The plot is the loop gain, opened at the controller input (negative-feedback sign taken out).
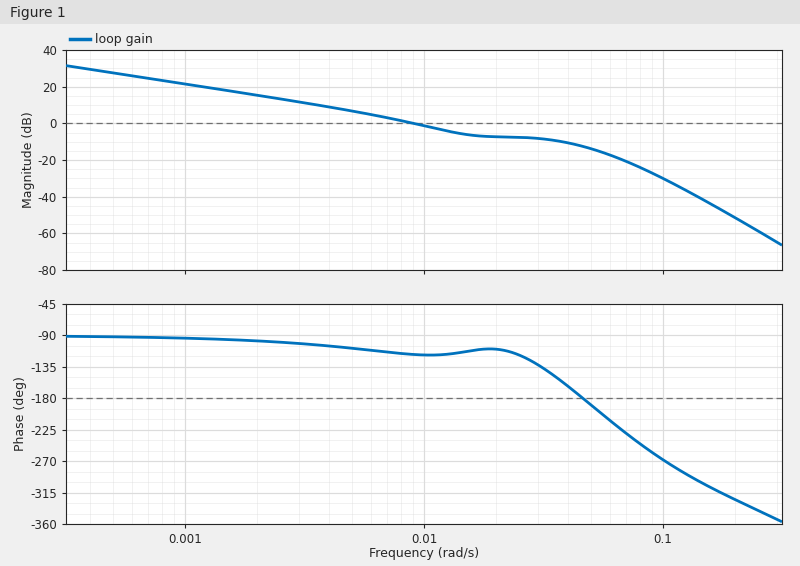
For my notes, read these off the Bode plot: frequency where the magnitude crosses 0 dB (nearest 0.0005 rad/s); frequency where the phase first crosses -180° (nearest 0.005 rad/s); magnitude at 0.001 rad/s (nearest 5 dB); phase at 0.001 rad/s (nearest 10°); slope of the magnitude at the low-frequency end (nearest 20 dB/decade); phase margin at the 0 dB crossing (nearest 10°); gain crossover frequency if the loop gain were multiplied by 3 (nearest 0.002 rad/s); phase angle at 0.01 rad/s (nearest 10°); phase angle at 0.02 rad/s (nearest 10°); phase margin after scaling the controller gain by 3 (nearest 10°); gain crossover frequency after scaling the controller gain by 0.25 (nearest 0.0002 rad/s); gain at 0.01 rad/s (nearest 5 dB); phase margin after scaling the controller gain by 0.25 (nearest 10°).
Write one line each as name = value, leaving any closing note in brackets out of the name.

frequency where the magnitude crosses 0 dB = 0.0090 rad/s
frequency where the phase first crosses -180° = 0.045 rad/s
magnitude at 0.001 rad/s = 20 dB
phase at 0.001 rad/s = -90°
slope of the magnitude at the low-frequency end = -20 dB/decade
phase margin at the 0 dB crossing = 60°
gain crossover frequency if the loop gain were multiplied by 3 = 0.036 rad/s
phase angle at 0.01 rad/s = -120°
phase angle at 0.02 rad/s = -110°
phase margin after scaling the controller gain by 3 = 30°
gain crossover frequency after scaling the controller gain by 0.25 = 0.0028 rad/s
gain at 0.01 rad/s = 0 dB
phase margin after scaling the controller gain by 0.25 = 80°
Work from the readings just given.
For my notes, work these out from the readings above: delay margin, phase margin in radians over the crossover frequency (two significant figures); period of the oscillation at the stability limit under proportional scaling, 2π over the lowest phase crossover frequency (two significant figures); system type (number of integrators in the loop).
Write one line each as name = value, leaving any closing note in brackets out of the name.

delay margin, phase margin in radians over the crossover frequency = 120 s
period of the oscillation at the stability limit under proportional scaling, 2π over the lowest phase crossover frequency = 140 s
system type = 1
